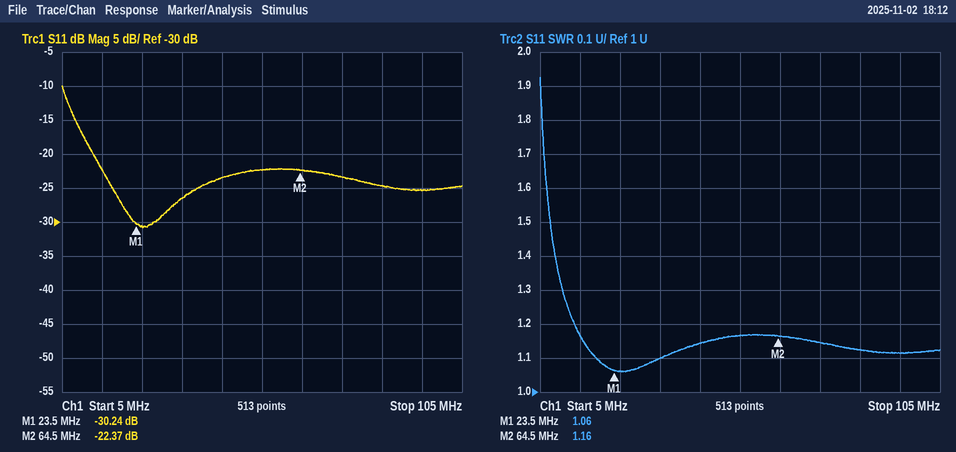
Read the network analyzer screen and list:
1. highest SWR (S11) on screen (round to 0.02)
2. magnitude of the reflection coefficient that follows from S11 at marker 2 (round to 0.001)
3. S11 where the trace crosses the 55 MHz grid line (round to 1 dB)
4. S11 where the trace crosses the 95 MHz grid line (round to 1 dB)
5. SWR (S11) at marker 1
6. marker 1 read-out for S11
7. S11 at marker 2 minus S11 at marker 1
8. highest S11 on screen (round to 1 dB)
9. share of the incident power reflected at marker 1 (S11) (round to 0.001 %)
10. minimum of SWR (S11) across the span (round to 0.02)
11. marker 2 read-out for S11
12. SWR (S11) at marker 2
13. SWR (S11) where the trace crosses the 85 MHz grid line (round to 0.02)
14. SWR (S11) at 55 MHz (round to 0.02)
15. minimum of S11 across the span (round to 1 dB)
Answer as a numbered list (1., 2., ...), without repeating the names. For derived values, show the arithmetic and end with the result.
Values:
1. 1.92
2. 10^(-22.37/20) ≈ 0.076
3. -22 dB
4. -25 dB
5. 1.06
6. -30.24 dB
7. -22.37 − (-30.24) = 7.87 dB
8. -10 dB
9. 10^(-30.24/10) ≈ 0.095 %
10. 1.06
11. -22.37 dB
12. 1.16
13. 1.12
14. 1.16
15. -31 dB
